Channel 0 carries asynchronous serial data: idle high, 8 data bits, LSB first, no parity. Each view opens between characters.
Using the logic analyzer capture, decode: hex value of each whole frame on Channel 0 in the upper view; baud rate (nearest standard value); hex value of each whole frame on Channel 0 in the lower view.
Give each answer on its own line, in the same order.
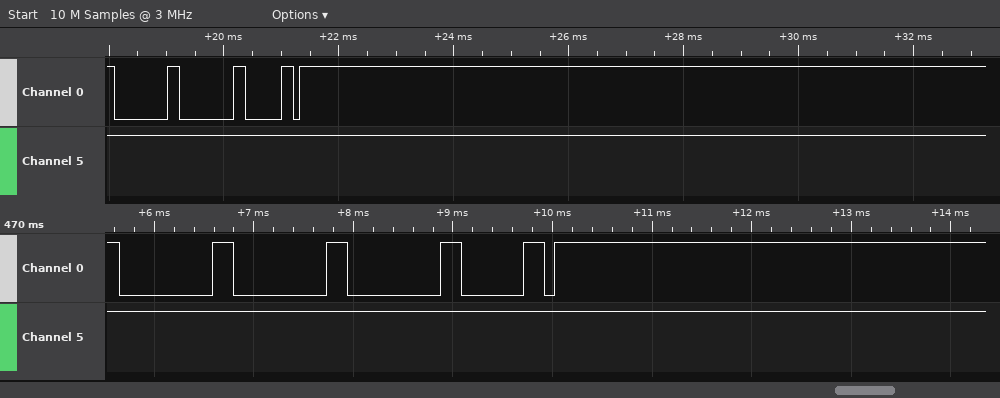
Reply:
00, 00, 60
9600 baud
00, 00, 00, 60
